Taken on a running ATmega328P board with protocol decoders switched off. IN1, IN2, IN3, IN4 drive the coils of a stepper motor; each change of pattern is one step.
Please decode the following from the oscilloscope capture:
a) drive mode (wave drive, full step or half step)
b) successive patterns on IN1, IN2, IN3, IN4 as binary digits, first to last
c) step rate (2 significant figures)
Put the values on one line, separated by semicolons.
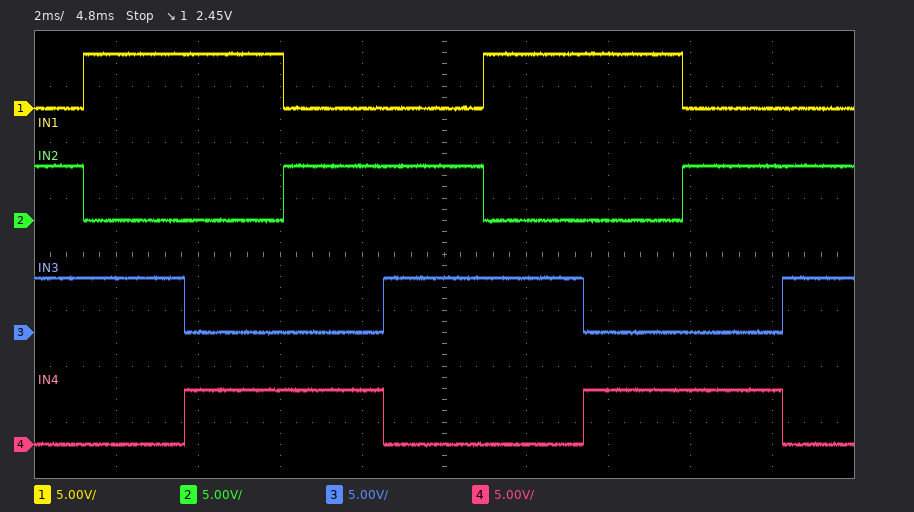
full step; 0110 1010 1001 0101 0110 1010 1001 0101 0110; 410 steps/s
